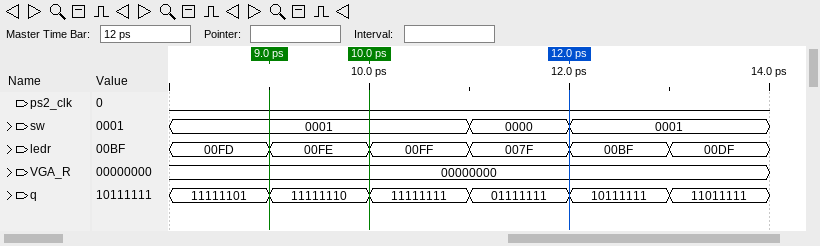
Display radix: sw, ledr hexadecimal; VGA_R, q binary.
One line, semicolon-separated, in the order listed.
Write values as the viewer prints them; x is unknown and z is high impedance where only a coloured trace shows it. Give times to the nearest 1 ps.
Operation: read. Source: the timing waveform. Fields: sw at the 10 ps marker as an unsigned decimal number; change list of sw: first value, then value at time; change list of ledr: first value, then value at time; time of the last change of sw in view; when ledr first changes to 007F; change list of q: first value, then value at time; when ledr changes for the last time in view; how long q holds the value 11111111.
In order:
1; 0001, 0000 at 11 ps, 0001 at 12 ps; 00FD, 00FE at 9 ps, 00FF at 10 ps, 007F at 11 ps, 00BF at 12 ps, 00DF at 13 ps; 12 ps; 11 ps; 11111101, 11111110 at 9 ps, 11111111 at 10 ps, 01111111 at 11 ps, 10111111 at 12 ps, 11011111 at 13 ps; 13 ps; 1 ps
